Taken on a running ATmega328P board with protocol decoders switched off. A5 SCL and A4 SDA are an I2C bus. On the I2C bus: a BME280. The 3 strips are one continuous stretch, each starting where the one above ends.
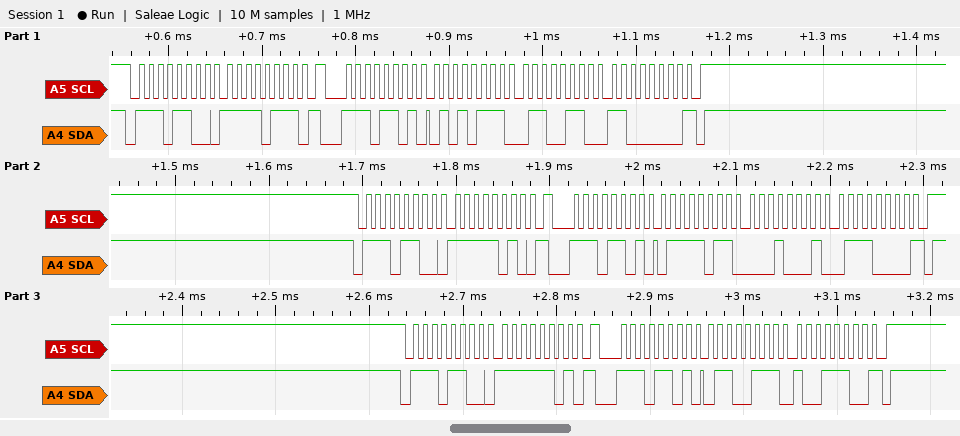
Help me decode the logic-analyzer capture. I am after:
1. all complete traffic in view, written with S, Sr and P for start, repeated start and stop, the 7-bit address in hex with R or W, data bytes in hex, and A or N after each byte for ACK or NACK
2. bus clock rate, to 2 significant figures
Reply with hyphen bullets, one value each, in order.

- S 76W A F7 A Sr 76R A 57 A 66 A C0 N P S 76W A FA A Sr 76R A 7B A 11 A 70 N P S 76W A FD A Sr 76R A 67 A 9C N P
- 100 kHz
